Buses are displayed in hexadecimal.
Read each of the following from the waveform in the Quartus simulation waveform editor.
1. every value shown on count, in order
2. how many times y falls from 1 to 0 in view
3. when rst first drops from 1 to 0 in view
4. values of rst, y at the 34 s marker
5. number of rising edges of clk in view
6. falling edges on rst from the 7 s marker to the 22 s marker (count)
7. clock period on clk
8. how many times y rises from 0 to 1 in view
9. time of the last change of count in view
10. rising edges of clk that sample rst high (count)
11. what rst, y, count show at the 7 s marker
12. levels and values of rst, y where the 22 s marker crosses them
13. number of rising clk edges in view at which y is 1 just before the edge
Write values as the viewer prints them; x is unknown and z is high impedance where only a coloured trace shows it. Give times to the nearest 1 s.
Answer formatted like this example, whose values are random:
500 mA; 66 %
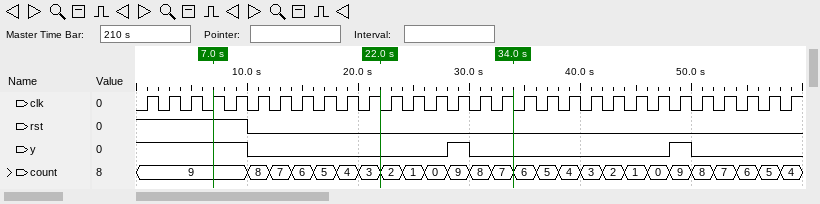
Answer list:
9, 8, 7, 6, 5, 4, 3, 2, 1, 0, 9, 8, 7, 6, 5, 4, 3, 2, 1, 0, 9, 8, 7, 6, 5, 4; 3; 10 s; rst=0, y=0; 30; 1; 2 s; 2; 58 s; 5; rst=1, y=1, count=9; rst=0, y=0; 7
